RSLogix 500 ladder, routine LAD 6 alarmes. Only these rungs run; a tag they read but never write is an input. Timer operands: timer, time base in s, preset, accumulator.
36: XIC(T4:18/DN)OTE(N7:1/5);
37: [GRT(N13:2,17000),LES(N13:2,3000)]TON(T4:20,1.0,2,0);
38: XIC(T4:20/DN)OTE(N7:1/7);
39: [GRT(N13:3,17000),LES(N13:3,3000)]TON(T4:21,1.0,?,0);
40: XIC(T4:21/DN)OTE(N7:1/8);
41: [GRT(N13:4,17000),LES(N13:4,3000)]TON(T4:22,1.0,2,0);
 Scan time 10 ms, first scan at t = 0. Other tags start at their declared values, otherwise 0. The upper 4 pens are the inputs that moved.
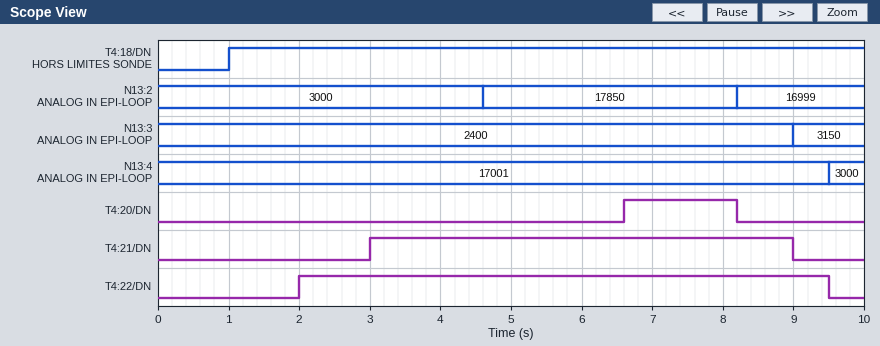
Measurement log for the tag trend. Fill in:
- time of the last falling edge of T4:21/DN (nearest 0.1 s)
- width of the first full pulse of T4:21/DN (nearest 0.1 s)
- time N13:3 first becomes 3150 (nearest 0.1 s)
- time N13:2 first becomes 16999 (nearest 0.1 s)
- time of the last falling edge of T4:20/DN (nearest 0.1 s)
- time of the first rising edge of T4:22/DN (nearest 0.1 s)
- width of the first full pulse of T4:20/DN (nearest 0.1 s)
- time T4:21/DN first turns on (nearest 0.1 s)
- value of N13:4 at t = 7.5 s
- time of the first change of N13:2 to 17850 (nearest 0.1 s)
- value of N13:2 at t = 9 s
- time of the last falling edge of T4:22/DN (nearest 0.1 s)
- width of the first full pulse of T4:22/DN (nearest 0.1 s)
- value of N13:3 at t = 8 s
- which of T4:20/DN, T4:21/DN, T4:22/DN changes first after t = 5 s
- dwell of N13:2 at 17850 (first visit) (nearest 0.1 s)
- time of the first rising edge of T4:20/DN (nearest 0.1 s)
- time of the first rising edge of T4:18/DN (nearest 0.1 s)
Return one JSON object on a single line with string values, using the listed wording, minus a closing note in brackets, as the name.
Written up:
{"time of the last falling edge of T4:21/DN": "9.0 s", "width of the first full pulse of T4:21/DN": "6.0 s", "time N13:3 first becomes 3150": "9.0 s", "time N13:2 first becomes 16999": "8.2 s", "time of the last falling edge of T4:20/DN": "8.2 s", "time of the first rising edge of T4:22/DN": "2.0 s", "width of the first full pulse of T4:20/DN": "1.6 s", "time T4:21/DN first turns on": "3.0 s", "value of N13:4 at t = 7.5 s": "17001", "time of the first change of N13:2 to 17850": "4.6 s", "value of N13:2 at t = 9 s": "16999", "time of the last falling edge of T4:22/DN": "9.5 s", "width of the first full pulse of T4:22/DN": "7.5 s", "value of N13:3 at t = 8 s": "2400", "which of T4:20/DN, T4:21/DN, T4:22/DN changes first after t = 5 s": "T4:20/DN", "dwell of N13:2 at 17850 (first visit)": "3.6 s", "time of the first rising edge of T4:20/DN": "6.6 s", "time of the first rising edge of T4:18/DN": "1.0 s"}
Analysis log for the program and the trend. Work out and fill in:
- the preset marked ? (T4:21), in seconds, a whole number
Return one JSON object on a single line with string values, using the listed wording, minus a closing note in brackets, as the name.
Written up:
{"the preset marked ? (T4:21), in seconds, a whole number": "3 s"}
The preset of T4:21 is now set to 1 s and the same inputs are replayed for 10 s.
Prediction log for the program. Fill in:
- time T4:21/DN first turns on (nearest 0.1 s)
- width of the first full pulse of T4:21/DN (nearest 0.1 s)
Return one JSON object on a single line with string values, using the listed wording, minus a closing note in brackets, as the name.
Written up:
{"time T4:21/DN first turns on": "1.0 s", "width of the first full pulse of T4:21/DN": "8.0 s"}
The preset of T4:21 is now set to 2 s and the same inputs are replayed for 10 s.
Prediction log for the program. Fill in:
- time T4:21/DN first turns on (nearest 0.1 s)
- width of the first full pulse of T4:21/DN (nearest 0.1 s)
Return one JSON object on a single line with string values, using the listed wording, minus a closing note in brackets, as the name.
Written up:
{"time T4:21/DN first turns on": "2.0 s", "width of the first full pulse of T4:21/DN": "7.0 s"}
